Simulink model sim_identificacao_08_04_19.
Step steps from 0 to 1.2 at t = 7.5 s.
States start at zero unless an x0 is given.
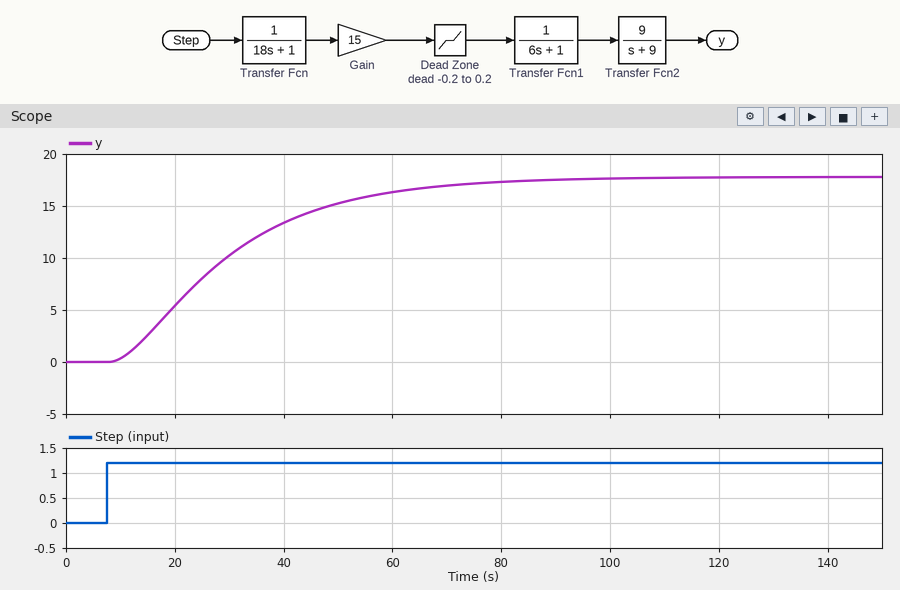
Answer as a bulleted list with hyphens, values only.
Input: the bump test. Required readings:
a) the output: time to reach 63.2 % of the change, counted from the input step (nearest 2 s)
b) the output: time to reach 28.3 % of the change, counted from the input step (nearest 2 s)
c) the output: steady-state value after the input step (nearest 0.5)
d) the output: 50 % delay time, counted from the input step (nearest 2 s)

- 26 s
- 12 s
- 18.0
- 20 s
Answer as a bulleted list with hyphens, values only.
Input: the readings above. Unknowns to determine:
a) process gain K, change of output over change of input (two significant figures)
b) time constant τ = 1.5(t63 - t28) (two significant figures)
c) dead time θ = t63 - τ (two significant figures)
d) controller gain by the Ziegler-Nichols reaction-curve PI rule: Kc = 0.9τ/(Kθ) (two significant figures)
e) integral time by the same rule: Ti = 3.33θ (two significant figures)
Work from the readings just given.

- 15
- 21 s
- 5.0 s
- 0.25
- 17 s
